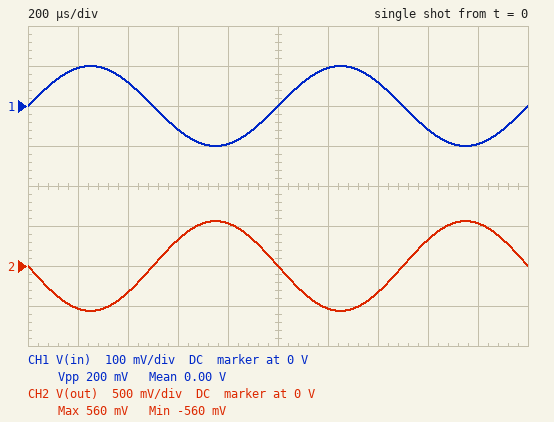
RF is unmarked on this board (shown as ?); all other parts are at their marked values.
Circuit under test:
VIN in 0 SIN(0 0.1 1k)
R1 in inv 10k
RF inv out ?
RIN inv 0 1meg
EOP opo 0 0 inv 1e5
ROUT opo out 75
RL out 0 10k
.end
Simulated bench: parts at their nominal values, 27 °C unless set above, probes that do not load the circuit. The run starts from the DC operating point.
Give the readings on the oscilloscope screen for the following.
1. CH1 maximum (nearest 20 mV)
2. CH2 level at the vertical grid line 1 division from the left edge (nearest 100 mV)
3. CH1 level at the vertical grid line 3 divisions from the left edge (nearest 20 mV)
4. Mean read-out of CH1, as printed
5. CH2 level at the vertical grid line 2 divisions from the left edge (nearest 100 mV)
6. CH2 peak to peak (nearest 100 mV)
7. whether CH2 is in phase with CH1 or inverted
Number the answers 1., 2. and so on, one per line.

1. 100 mV
2. -500 mV
3. -60 mV
4. 0.00 V
5. -300 mV
6. 1.1 V
7. inverted
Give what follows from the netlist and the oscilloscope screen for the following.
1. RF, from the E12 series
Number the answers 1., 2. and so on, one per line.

1. 56 kΩ
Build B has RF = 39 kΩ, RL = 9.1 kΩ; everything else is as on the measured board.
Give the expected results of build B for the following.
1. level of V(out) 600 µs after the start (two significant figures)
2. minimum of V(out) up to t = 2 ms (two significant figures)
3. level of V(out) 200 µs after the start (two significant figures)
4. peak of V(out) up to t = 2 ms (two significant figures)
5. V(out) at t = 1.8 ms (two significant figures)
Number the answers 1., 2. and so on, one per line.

1. 230 mV
2. -390 mV
3. -370 mV
4. 390 mV
5. 370 mV
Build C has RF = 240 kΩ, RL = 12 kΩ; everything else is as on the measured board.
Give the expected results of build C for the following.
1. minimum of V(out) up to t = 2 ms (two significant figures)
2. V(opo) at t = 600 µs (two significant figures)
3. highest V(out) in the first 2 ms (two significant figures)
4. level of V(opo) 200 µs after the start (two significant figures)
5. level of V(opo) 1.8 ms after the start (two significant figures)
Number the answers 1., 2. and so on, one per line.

1. -2.4 V
2. 1.4 V
3. 2.4 V
4. -2.3 V
5. 2.3 V
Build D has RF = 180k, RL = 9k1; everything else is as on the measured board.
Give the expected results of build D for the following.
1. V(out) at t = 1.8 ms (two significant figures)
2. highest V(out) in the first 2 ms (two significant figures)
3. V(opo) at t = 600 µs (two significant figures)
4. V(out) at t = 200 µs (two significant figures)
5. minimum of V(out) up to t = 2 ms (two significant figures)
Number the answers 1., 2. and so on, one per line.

1. 1.7 V
2. 1.8 V
3. 1.1 V
4. -1.7 V
5. -1.8 V
